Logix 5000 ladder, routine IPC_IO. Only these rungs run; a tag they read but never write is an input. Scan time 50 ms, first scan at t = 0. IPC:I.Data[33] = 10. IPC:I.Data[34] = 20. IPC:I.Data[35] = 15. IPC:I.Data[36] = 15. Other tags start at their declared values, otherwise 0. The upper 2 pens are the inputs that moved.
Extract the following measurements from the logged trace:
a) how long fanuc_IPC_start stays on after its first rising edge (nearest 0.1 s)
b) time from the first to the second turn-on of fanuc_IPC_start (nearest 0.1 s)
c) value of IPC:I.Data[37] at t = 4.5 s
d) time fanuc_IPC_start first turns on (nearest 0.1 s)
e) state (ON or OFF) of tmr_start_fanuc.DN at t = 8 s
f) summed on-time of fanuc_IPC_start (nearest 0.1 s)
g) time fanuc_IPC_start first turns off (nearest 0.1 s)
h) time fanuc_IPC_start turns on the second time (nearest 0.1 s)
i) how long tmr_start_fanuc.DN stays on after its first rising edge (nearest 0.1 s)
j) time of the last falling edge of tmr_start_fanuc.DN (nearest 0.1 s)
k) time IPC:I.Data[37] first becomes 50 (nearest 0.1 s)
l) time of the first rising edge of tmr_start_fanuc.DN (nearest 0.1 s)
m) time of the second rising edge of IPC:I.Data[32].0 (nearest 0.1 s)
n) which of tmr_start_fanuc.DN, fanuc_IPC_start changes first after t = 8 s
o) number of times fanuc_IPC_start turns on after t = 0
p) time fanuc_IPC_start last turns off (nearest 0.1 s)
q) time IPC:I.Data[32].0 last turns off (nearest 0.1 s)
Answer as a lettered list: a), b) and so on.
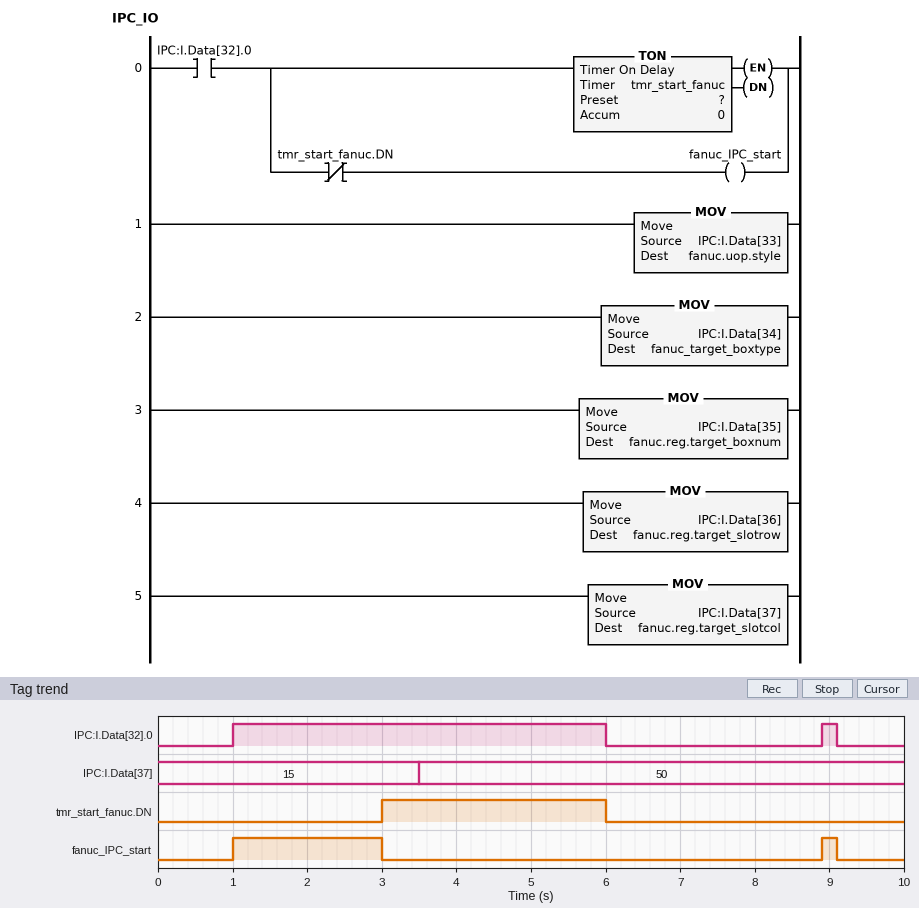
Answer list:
a) 2.0 s
b) 7.9 s
c) 50
d) 1.0 s
e) OFF
f) 2.2 s
g) 3.0 s
h) 8.9 s
i) 3.0 s
j) 6.0 s
k) 3.5 s
l) 3.0 s
m) 8.9 s
n) fanuc_IPC_start
o) 2
p) 9.1 s
q) 9.1 s
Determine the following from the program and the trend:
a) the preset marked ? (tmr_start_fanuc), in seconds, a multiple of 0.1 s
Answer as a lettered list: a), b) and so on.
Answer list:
a) 2.0 s
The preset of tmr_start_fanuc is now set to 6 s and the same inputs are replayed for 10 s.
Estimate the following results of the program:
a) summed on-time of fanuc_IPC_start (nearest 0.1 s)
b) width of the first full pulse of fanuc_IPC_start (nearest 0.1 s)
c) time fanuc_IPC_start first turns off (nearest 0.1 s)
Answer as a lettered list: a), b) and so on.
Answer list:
a) 5.2 s
b) 5.0 s
c) 6.0 s
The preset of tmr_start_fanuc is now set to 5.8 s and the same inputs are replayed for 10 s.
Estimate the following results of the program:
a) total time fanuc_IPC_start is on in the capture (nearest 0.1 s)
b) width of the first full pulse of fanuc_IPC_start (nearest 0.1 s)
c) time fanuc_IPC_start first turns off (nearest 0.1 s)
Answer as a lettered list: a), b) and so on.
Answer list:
a) 5.2 s
b) 5.0 s
c) 6.0 s
